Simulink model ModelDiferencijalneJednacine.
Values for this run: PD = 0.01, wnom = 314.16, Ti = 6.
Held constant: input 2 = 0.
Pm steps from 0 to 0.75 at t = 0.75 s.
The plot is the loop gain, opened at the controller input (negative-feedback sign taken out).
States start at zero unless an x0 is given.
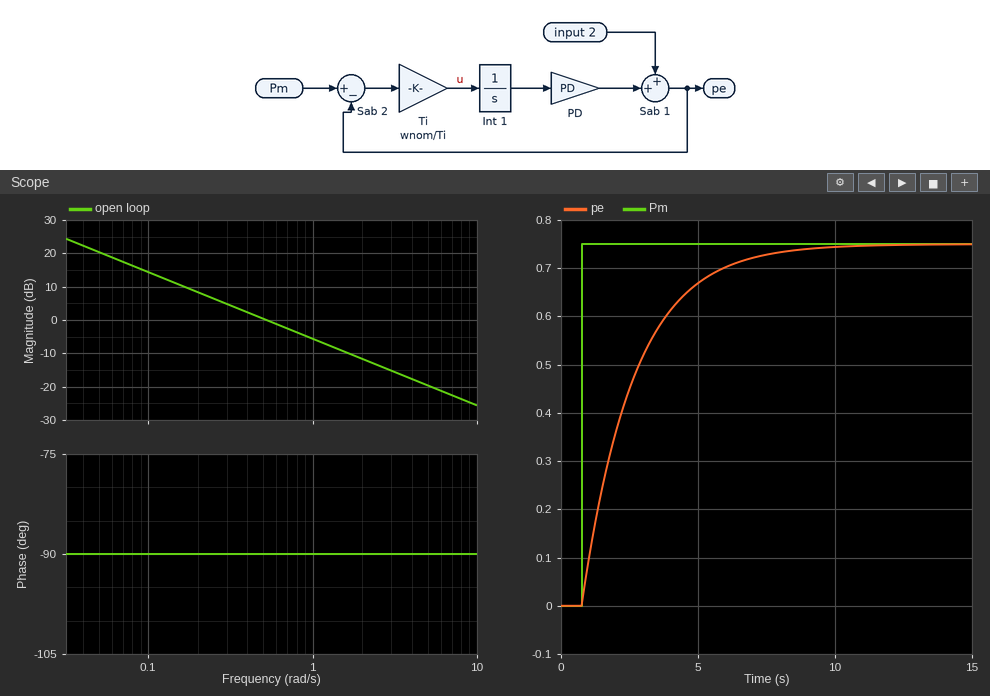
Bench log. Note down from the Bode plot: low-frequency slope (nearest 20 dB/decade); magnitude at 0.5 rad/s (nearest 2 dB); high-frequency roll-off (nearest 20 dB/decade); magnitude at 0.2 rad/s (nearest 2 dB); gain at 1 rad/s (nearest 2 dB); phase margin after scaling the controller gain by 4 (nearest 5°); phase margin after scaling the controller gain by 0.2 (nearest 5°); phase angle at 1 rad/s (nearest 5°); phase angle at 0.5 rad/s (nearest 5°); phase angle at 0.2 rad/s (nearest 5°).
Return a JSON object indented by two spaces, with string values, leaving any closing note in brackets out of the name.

{
  "low-frequency slope": "-20 dB/decade",
  "magnitude at 0.5 rad/s": "0 dB",
  "high-frequency roll-off": "-20 dB/decade",
  "magnitude at 0.2 rad/s": "8 dB",
  "gain at 1 rad/s": "-6 dB",
  "phase margin after scaling the controller gain by 4": "90°",
  "phase margin after scaling the controller gain by 0.2": "90°",
  "phase angle at 1 rad/s": "-90°",
  "phase angle at 0.5 rad/s": "-90°",
  "phase angle at 0.2 rad/s": "-90°"
}
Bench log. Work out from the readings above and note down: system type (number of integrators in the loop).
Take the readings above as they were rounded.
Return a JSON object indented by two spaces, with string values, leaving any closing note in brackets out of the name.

{
  "system type": "1"
}
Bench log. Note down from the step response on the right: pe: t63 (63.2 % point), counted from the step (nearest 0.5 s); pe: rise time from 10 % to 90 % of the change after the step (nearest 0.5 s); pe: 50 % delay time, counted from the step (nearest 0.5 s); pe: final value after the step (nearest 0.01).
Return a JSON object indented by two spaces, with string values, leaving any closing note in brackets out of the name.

{
  "pe: t63 (63.2 % point), counted from the step": "2.0 s",
  "pe: rise time from 10 % to 90 % of the change after the step": "4.0 s",
  "pe: 50 % delay time, counted from the step": "1.5 s",
  "pe: final value after the step": "0.75"
}
